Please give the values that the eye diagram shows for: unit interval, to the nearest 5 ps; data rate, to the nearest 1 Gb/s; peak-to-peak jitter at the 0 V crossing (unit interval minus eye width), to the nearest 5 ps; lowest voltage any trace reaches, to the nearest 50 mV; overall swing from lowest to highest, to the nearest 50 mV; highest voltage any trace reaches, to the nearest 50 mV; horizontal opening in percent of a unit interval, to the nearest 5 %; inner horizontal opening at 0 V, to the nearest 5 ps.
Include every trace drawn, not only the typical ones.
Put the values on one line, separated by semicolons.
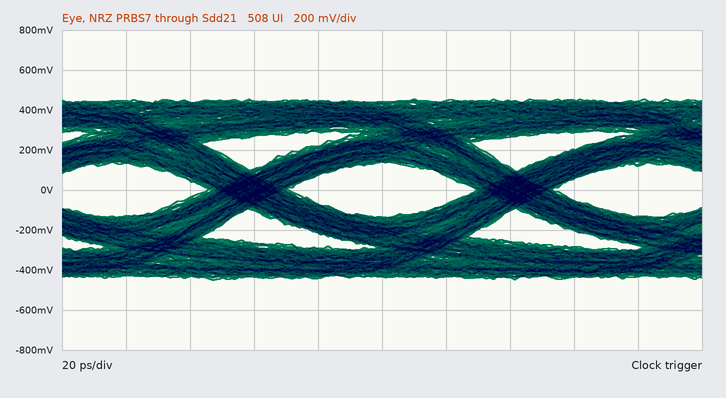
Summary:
85 ps; 12 Gb/s; 25 ps; -450 mV; 900 mV; 450 mV; 70 %; 60 ps
